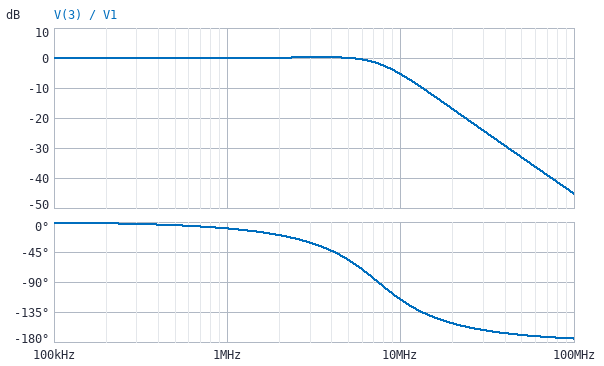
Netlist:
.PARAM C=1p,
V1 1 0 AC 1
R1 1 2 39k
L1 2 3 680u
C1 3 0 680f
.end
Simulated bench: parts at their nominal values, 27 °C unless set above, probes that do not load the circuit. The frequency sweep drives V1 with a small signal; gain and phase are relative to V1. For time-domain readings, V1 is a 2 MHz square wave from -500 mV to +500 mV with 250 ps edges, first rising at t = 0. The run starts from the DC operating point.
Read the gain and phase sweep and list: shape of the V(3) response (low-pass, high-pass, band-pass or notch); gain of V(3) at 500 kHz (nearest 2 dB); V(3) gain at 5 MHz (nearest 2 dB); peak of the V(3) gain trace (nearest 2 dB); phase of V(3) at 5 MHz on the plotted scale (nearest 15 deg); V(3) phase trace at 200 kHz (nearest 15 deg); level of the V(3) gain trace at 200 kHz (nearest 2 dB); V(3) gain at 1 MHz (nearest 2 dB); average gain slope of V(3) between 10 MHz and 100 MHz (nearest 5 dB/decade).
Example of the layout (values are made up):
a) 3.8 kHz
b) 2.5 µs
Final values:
a) low-pass
b) 0 dB
c) 0 dB
d) 0 dB
e) -60 deg
f) 0 deg
g) 0 dB
h) 0 dB
i) -40 dB/decade
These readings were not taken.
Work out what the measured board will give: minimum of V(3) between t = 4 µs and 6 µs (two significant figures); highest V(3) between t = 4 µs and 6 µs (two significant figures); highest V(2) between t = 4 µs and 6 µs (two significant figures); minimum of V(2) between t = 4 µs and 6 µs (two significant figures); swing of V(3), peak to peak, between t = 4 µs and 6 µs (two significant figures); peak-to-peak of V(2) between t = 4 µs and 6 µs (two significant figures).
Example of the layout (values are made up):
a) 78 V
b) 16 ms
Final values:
a) -590 mV
b) 590 mV
c) 550 mV
d) -550 mV
e) 1.2 V
f) 1.1 V
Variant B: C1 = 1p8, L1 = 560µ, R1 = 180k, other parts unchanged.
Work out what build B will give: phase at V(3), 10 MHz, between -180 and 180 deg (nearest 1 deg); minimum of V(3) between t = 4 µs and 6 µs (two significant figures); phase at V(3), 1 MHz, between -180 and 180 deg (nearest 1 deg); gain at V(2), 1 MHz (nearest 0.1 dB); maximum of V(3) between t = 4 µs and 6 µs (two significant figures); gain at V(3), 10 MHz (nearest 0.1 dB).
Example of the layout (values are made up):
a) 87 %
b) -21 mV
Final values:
a) -98 deg
b) -180 mV
c) -65 deg
d) -7.4 dB
e) 180 mV
f) -26.3 dB
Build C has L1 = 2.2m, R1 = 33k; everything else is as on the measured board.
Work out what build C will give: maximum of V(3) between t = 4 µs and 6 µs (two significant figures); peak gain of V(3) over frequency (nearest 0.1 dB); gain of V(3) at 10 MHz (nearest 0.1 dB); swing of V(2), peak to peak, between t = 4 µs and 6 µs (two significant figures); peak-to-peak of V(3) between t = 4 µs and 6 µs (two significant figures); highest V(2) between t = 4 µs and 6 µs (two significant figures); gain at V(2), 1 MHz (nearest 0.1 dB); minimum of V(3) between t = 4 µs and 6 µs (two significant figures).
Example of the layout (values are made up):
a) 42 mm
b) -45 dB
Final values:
a) 840 mV
b) 5.1 dB
c) -14.2 dB
d) 1.3 V
e) 1.7 V
f) 630 mV
g) -0.1 dB
h) -840 mV
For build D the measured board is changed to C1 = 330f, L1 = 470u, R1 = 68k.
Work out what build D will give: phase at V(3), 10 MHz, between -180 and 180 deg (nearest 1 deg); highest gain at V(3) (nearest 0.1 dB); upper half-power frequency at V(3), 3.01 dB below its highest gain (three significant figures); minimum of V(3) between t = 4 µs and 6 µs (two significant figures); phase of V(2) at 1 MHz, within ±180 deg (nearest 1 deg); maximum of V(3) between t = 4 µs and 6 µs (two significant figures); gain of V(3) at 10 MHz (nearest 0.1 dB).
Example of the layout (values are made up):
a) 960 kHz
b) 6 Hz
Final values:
a) -75 deg
b) 0 dB
c) 9.52 MHz
d) -500 mV
e) -8 deg
f) 500 mV
g) -3.3 dB
